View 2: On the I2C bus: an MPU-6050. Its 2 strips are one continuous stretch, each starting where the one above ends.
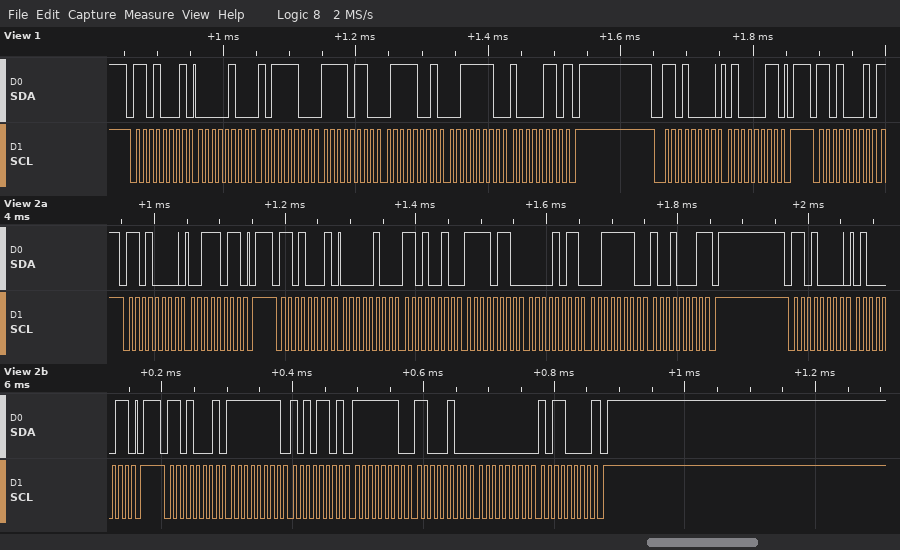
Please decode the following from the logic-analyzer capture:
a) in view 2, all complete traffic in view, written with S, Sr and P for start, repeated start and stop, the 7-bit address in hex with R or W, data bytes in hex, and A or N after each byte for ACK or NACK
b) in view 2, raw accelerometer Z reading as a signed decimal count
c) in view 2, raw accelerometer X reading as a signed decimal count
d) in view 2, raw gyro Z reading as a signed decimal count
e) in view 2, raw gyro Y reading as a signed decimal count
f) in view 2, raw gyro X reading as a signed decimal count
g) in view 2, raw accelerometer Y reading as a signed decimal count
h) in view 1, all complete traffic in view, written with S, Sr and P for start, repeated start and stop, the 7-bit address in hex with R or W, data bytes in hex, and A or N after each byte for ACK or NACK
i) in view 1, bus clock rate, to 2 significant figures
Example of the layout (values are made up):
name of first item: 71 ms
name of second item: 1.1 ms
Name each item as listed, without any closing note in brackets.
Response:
in view 2, all complete traffic in view, written with S, Sr and P for start, repeated start and stop, the 7-bit address in hex with R or W, data bytes in hex, and A or N after each byte for ACK or NACK: S 68W A 3B A P S 68R A 04 A D2 A F6 A 0B A 3E A 91 N P S 68W A 43 A P S 68R A FF A AD A FE A C4 A 00 A B0 N P
in view 2, raw accelerometer Z reading as a signed decimal count: 16017
in view 2, raw accelerometer X reading as a signed decimal count: 1234
in view 2, raw gyro Z reading as a signed decimal count: 176
in view 2, raw gyro Y reading as a signed decimal count: -316
in view 2, raw gyro X reading as a signed decimal count: -83
in view 2, raw accelerometer Y reading as a signed decimal count: -2549
in view 1, all complete traffic in view, written with S, Sr and P for start, repeated start and stop, the 7-bit address in hex with R or W, data bytes in hex, and A or N after each byte for ACK or NACK: S 68R A 04 A BC A F6 A 79 A 3E A 86 N P S 68W A 43 A P S 68R A
in view 1, bus clock rate, to 2 significant figures: 100 kHz
